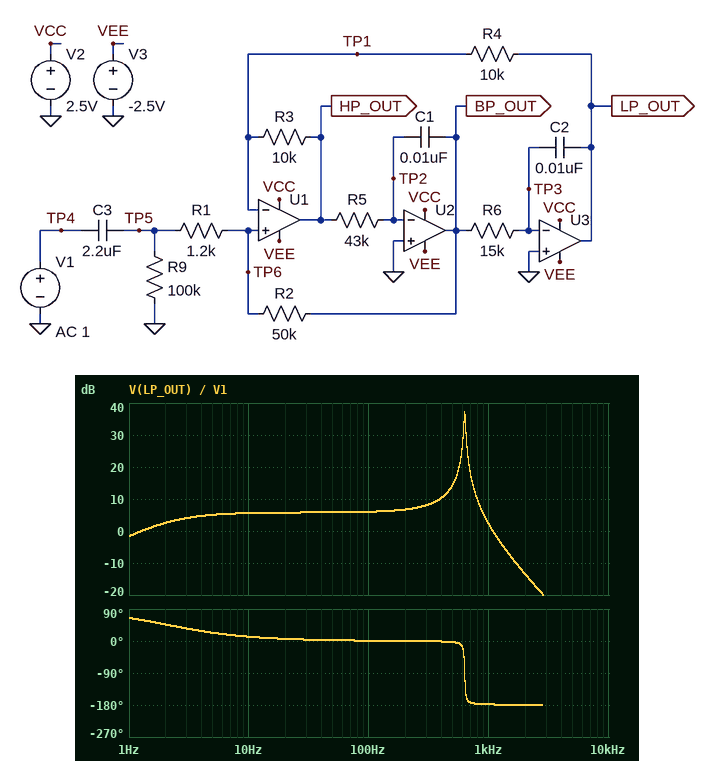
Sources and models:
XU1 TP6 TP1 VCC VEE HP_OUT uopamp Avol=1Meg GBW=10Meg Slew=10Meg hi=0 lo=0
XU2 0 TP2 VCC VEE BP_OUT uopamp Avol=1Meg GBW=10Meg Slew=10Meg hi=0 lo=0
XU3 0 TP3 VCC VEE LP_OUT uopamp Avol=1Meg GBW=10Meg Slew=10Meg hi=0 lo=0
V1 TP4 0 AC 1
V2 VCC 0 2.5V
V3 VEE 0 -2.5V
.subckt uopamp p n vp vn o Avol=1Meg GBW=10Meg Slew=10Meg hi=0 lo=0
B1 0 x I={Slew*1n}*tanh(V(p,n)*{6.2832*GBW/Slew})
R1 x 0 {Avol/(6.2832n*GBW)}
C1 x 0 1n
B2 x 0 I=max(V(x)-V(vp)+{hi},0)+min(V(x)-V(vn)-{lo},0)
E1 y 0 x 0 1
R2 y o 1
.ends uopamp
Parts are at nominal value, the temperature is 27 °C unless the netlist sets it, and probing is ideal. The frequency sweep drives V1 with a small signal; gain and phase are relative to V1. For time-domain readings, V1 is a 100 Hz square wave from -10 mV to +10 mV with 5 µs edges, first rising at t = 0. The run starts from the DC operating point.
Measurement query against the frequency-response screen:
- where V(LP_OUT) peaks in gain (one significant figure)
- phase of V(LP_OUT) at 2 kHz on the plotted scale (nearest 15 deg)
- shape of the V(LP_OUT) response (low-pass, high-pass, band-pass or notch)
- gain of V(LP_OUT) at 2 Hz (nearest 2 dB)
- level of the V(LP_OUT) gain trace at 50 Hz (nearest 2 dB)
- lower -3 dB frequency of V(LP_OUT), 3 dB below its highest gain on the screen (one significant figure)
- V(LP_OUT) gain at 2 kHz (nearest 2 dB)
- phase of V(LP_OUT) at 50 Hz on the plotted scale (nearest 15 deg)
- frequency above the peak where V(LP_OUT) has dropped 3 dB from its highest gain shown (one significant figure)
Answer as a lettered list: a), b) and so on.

a) 600 Hz
b) -180 deg
c) band-pass
d) 2 dB
e) 6 dB
f) 600 Hz
g) -14 dB
h) 0 deg
i) 600 Hz
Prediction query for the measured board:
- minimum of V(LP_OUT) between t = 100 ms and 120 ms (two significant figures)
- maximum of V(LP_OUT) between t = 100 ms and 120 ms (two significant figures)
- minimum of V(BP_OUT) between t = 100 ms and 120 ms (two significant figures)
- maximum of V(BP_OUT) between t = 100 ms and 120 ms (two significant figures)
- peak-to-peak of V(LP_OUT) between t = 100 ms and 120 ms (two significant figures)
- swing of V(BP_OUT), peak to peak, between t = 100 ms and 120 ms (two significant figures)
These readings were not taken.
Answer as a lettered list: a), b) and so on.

a) -39 mV
b) 48 mV
c) -14 mV
d) 14 mV
e) 87 mV
f) 28 mV
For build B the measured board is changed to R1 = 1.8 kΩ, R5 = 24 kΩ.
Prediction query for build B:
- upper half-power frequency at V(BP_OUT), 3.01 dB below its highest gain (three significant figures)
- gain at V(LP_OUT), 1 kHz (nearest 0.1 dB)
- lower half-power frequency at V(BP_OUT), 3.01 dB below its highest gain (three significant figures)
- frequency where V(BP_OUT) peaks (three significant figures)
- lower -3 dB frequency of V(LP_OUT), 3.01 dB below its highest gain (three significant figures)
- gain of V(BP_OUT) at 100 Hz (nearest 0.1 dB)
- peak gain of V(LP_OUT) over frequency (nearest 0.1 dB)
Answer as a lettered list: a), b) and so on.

a) 863 Hz
b) 13.2 dB
c) 817 Hz
d) 840 Hz
e) 816 Hz
f) -14.7 dB
g) 31.0 dB
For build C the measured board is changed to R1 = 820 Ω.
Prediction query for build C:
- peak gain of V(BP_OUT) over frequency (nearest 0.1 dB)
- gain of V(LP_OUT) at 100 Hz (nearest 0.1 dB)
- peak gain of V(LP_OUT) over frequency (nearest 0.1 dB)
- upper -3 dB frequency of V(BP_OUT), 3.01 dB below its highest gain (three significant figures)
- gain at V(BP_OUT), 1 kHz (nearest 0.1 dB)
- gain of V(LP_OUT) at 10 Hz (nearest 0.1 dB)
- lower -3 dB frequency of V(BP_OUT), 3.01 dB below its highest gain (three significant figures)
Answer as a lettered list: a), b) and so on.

a) 35.8 dB
b) 6.1 dB
c) 40.4 dB
d) 633 Hz
e) 1.6 dB
f) 5.7 dB
g) 622 Hz
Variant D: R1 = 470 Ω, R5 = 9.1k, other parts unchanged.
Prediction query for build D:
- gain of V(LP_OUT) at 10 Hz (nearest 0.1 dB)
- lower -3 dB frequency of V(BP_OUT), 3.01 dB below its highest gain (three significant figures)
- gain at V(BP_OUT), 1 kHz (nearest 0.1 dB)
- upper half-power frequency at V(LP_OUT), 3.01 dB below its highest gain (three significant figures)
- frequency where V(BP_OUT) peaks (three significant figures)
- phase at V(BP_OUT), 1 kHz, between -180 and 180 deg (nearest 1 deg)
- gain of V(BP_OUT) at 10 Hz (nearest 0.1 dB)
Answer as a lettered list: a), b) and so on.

a) 5.7 dB
b) 1.35 kHz
c) 12.1 dB
d) 1.38 kHz
e) 1.36 kHz
f) -92 deg
g) -34.8 dB
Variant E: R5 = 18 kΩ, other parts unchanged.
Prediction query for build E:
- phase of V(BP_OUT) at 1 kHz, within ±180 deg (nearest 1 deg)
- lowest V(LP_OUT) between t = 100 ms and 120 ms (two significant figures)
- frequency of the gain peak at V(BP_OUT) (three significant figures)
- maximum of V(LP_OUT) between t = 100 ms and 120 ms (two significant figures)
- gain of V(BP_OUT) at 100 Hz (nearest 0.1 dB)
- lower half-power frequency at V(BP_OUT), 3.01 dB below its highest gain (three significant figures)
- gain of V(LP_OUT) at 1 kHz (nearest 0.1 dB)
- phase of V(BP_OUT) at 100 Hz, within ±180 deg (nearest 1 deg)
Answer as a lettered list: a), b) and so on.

a) 125 deg
b) -43 mV
c) 970 Hz
d) 52 mV
e) -14.6 dB
f) 949 Hz
g) 28.1 dB
h) -89 deg
